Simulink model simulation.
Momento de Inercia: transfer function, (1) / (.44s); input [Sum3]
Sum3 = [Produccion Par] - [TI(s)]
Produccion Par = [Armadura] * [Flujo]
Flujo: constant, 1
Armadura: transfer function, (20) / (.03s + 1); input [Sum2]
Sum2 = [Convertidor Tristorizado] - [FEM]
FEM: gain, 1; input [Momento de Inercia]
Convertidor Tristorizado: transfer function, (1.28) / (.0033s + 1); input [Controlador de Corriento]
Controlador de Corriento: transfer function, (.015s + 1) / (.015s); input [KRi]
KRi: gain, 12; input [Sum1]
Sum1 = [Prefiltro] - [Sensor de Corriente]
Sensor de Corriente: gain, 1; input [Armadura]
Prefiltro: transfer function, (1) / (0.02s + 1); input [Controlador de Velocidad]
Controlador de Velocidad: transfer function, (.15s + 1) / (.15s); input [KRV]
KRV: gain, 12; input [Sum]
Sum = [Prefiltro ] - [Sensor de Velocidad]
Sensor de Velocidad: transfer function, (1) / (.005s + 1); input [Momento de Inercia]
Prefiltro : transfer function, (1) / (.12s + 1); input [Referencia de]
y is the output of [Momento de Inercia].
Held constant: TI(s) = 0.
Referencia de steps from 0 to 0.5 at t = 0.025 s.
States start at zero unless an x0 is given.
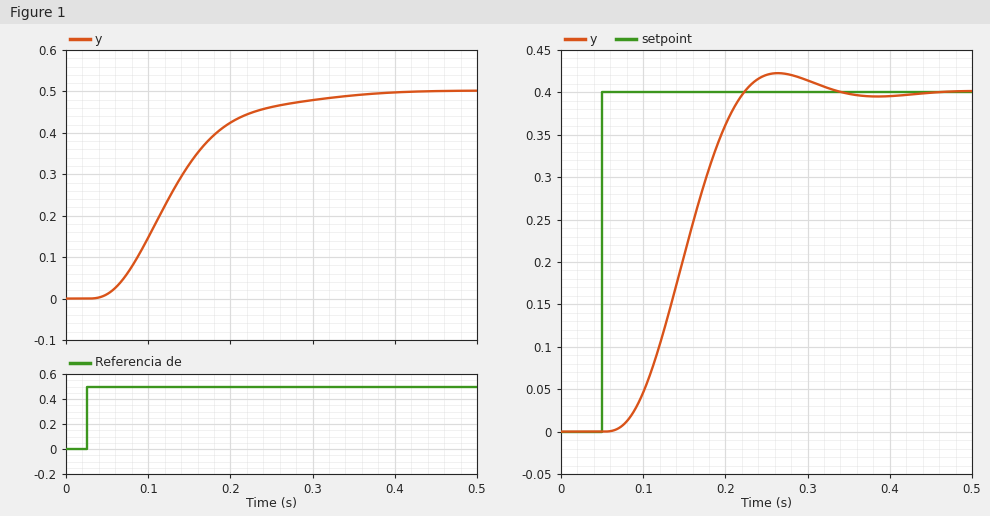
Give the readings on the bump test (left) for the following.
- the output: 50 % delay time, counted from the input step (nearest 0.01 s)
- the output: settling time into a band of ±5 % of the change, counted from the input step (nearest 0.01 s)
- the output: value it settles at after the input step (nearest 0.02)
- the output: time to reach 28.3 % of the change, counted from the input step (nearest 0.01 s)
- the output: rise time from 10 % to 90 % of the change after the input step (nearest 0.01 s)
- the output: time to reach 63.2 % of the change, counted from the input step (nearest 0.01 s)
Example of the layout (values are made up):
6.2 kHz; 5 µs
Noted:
0.10 s; 0.26 s; 0.50; 0.07 s; 0.16 s; 0.12 s
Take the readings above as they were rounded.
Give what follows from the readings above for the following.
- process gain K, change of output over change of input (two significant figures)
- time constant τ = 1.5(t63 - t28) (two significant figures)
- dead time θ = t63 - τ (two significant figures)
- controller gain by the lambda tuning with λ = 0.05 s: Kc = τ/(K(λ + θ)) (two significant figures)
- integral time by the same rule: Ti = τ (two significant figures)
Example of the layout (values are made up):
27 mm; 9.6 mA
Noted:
1.0; 0.075 s; 0.045 s; 0.79; 0.075 s
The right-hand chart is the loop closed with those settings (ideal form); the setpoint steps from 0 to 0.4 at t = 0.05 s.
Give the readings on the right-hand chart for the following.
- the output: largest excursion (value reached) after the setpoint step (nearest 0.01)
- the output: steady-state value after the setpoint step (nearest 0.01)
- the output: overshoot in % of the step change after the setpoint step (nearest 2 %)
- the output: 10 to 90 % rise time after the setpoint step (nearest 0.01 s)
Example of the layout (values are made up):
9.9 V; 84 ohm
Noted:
0.42; 0.40; 6 %; 0.10 s
